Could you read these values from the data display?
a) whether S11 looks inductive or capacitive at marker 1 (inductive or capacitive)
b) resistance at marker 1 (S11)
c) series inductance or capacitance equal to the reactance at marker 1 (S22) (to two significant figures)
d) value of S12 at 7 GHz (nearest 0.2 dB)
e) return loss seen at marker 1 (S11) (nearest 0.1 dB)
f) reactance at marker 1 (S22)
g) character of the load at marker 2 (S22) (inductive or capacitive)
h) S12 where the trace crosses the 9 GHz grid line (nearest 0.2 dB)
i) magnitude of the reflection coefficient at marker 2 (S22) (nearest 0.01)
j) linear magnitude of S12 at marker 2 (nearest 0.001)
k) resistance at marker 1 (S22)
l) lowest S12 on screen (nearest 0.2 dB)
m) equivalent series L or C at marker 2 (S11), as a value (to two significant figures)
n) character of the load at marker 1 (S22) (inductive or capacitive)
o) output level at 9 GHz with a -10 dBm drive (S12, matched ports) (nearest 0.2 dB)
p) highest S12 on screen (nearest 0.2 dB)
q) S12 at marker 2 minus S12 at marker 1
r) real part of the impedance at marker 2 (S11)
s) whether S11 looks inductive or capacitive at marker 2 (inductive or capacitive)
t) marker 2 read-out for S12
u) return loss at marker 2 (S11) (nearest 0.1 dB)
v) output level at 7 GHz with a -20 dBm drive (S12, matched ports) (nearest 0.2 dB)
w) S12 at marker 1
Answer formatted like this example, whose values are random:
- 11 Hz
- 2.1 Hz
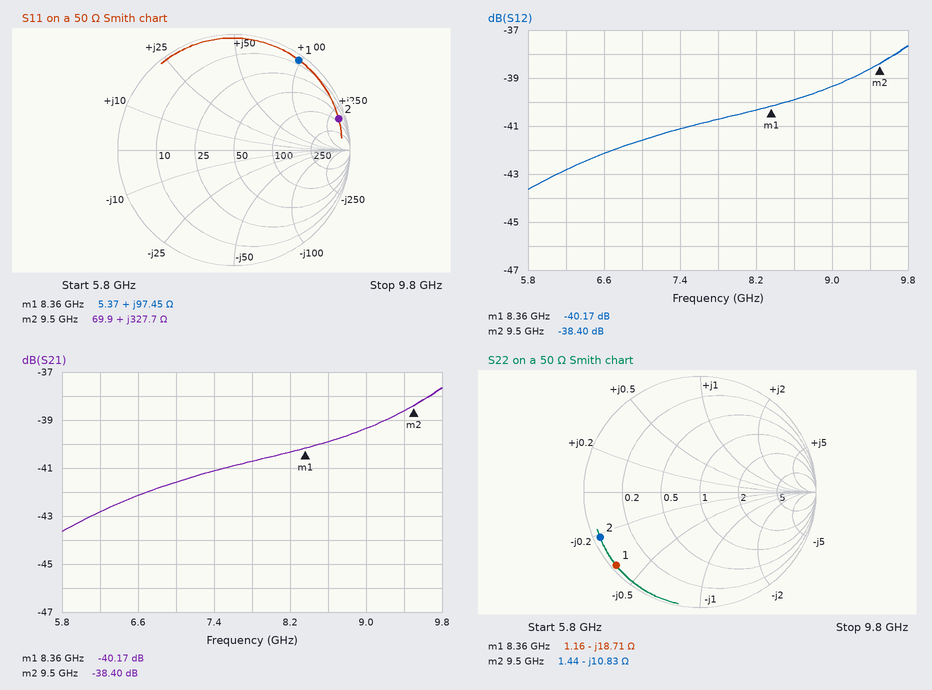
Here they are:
- inductive
- 5.37 Ω
- 1.0 pF
- -41.6 dB
- 0.4 dB
- -18.71 Ω
- capacitive
- -39.4 dB
- 0.95
- 0.012
- 1.16 Ω
- -43.6 dB
- 5.5 nH
- capacitive
- -49.4 dBm
- -37.6 dB
- 1.77 dB
- 69.9 Ω
- inductive
- -38.40 dB
- 0.5 dB
- -61.6 dBm
- -40.17 dB
